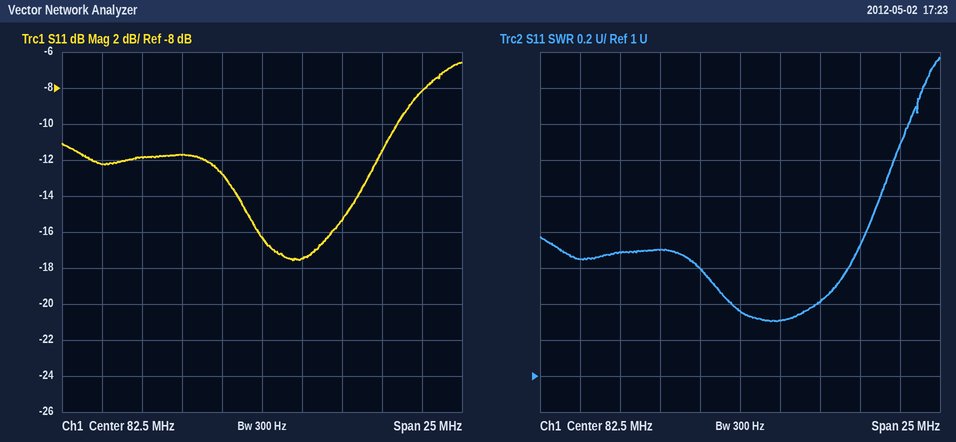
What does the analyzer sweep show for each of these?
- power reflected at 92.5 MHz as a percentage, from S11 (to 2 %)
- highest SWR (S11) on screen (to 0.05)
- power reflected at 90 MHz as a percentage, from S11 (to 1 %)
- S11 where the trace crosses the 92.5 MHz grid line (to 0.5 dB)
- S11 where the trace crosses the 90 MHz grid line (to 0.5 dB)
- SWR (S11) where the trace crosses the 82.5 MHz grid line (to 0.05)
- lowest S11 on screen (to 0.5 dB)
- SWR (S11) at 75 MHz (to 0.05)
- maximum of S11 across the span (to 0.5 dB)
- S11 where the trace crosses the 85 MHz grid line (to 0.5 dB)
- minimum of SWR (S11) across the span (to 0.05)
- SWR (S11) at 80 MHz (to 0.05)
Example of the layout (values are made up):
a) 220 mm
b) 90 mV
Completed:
a) 16 %
b) 2.75
c) 7 %
d) -8.0 dB
e) -11.5 dB
f) 1.35
g) -17.5 dB
h) 1.70
i) -6.5 dB
j) -17.5 dB
k) 1.30
l) 1.60
